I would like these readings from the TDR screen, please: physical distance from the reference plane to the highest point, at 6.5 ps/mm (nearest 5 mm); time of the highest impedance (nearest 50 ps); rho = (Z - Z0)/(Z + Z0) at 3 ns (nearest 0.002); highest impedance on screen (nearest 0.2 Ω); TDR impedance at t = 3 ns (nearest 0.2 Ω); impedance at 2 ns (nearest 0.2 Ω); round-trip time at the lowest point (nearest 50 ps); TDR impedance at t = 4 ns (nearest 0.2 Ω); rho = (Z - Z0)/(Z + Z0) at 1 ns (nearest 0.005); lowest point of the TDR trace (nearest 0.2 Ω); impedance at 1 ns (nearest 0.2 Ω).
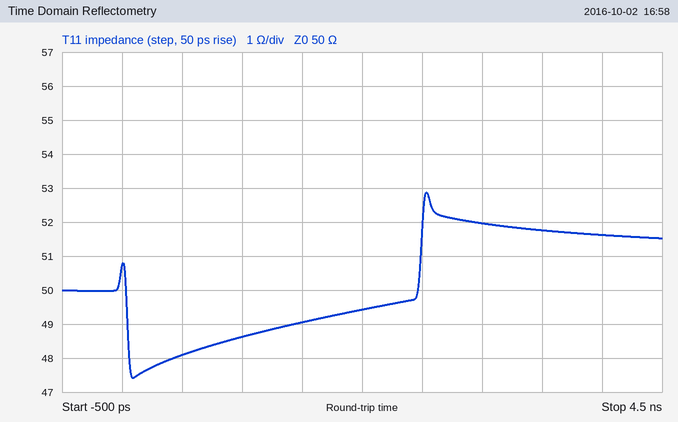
195 mm
2.55 ns
+0.020
52.8 Ω
52.0 Ω
49.4 Ω
100 ps
51.6 Ω
-0.015
47.4 Ω
48.6 Ω
